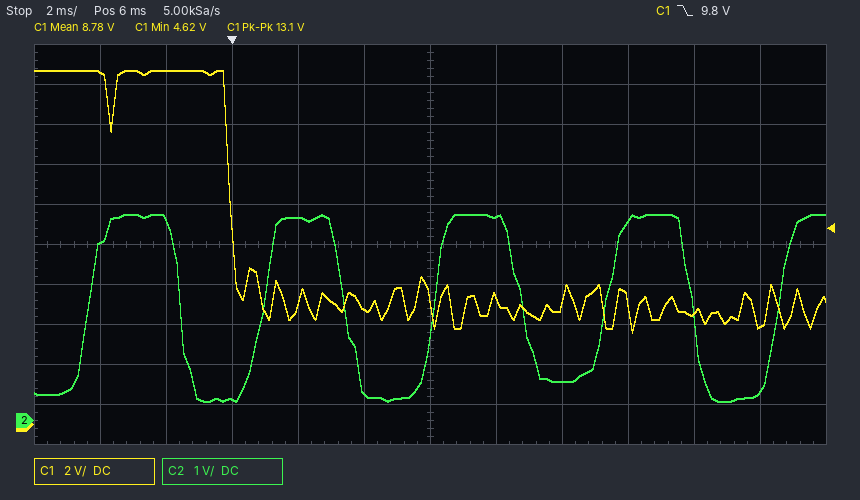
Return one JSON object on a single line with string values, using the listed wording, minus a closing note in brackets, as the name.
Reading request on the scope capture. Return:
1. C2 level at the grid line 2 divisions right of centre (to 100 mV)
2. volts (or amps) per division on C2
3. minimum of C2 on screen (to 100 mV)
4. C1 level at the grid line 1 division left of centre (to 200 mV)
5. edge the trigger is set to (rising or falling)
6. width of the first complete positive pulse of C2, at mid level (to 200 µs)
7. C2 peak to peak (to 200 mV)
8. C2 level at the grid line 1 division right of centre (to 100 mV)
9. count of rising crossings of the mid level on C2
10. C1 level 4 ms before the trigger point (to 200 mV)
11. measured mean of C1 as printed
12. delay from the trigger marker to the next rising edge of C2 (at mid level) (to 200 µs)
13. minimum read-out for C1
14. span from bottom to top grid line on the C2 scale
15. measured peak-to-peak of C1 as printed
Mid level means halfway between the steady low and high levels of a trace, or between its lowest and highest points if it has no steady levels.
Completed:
{"C2 level at the grid line 2 divisions right of centre": "1.0 V", "volts (or amps) per division on C2": "1 V", "minimum of C2 on screen": "500 mV", "C1 level at the grid line 1 division left of centre": "5.8 V", "edge the trigger is set to": "falling", "width of the first complete positive pulse of C2, at mid level": "2.8 ms", "C2 peak to peak": "4.6 V", "C2 level at the grid line 1 division right of centre": "5.1 V", "count of rising crossings of the mid level on C2": "5", "C1 level 4 ms before the trigger point": "17.6 V", "measured mean of C1 as printed": "8.78 V", "delay from the trigger marker to the next rising edge of C2 (at mid level)": "1.0 ms", "minimum read-out for C1": "4.62 V", "span from bottom to top grid line on the C2 scale": "10 V", "measured peak-to-peak of C1 as printed": "13.1 V"}
